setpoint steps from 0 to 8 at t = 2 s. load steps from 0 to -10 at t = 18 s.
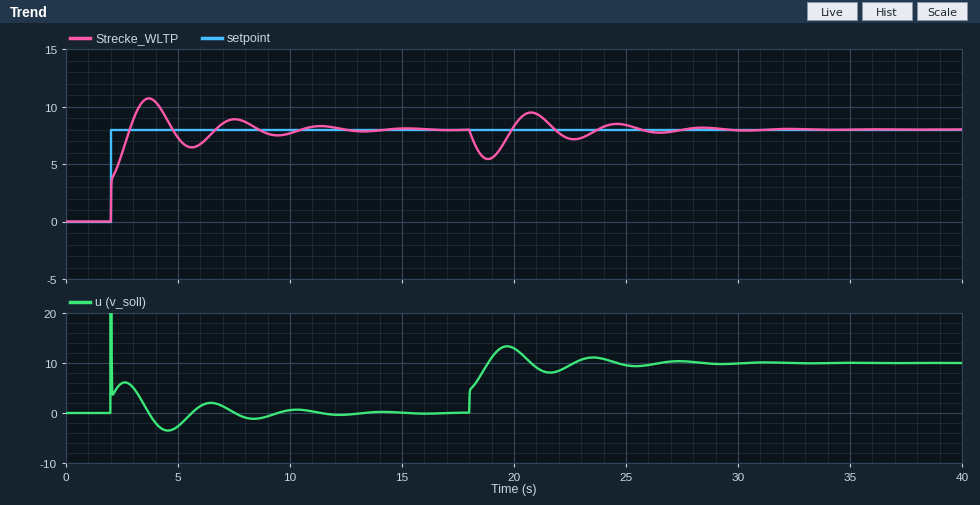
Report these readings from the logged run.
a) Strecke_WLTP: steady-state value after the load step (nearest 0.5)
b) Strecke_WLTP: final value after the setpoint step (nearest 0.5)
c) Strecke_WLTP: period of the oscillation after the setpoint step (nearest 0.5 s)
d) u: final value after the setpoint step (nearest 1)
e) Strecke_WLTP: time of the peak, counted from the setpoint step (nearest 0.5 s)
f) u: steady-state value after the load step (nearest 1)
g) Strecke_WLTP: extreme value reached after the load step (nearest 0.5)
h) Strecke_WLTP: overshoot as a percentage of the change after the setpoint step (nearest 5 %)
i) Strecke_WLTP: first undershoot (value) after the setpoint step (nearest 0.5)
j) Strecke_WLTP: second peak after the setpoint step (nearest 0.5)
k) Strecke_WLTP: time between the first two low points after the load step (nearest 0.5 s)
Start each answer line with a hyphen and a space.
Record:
- 8.0
- 8.0
- 4.0 s
- 0
- 1.5 s
- 10
- 5.5
- 35 %
- 6.5
- 9.0
- 4.0 s
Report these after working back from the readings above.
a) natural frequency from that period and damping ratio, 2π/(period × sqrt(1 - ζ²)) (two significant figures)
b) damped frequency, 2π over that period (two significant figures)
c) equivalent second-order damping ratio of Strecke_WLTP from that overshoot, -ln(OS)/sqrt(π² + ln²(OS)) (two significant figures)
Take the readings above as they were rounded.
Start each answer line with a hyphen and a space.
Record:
- 1.7 rad/s
- 1.6 rad/s
- 0.32
